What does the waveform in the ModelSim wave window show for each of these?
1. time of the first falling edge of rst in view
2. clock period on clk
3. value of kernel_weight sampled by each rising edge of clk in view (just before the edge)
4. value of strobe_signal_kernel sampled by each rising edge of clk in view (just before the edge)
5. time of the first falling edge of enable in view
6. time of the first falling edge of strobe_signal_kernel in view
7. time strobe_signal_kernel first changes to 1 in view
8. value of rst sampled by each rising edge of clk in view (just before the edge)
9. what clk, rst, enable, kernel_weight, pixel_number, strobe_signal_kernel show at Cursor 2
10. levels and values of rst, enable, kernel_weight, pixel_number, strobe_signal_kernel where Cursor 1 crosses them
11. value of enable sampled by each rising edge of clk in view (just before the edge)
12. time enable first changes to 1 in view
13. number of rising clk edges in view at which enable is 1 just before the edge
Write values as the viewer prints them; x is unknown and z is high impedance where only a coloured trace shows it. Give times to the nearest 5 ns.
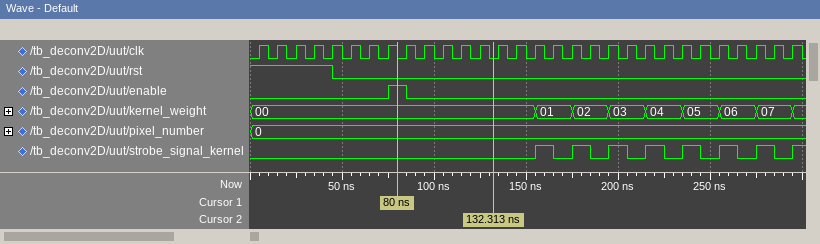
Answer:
45 ns
10 ns
00, 00, 00, 00, 00, 00, 00, 00, 00, 00, 00, 00, 00, 00, 00, 00, 01, 01, 02, 02, 03, 03, 04, 04, 05, 05, 06, 06, 07, 07
0 0 0 0 0 0 0 0 0 0 0 0 0 0 0 0 1 0 1 0 1 0 1 0 1 0 1 0 1 0
85 ns
165 ns
155 ns
1 1 1 1 1 0 0 0 0 0 0 0 0 0 0 0 0 0 0 0 0 0 0 0 0 0 0 0 0 0
clk=0, rst=0, enable=0, kernel_weight=00, pixel_number=0, strobe_signal_kernel=0
rst=0, enable=1, kernel_weight=00, pixel_number=0, strobe_signal_kernel=0
0 0 0 0 0 0 0 0 1 0 0 0 0 0 0 0 0 0 0 0 0 0 0 0 0 0 0 0 0 0
75 ns
1
